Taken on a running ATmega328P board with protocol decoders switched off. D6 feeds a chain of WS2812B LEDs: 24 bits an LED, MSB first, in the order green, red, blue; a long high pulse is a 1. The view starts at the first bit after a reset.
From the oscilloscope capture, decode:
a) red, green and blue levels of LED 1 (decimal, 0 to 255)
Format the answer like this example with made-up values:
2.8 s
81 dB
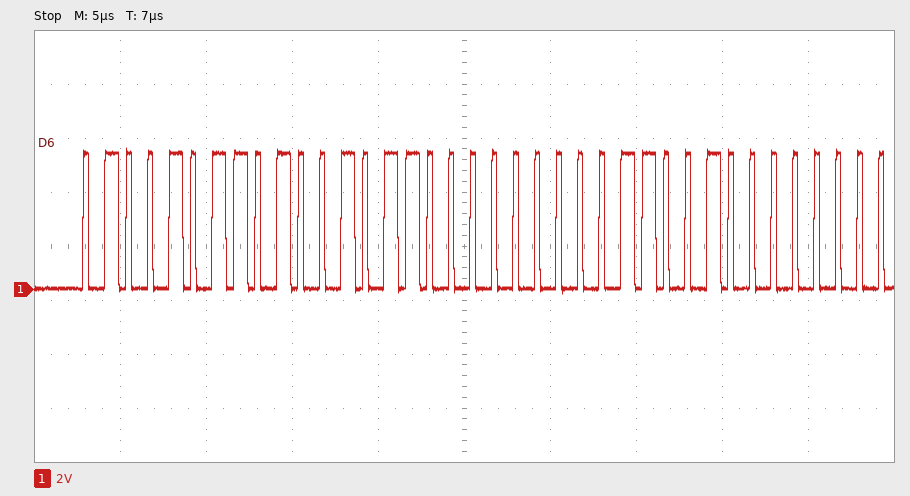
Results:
75, 75, 0
